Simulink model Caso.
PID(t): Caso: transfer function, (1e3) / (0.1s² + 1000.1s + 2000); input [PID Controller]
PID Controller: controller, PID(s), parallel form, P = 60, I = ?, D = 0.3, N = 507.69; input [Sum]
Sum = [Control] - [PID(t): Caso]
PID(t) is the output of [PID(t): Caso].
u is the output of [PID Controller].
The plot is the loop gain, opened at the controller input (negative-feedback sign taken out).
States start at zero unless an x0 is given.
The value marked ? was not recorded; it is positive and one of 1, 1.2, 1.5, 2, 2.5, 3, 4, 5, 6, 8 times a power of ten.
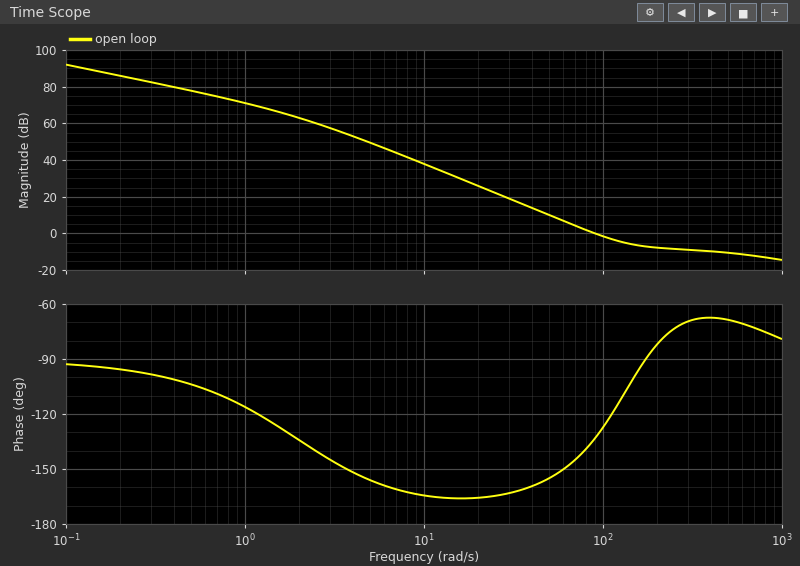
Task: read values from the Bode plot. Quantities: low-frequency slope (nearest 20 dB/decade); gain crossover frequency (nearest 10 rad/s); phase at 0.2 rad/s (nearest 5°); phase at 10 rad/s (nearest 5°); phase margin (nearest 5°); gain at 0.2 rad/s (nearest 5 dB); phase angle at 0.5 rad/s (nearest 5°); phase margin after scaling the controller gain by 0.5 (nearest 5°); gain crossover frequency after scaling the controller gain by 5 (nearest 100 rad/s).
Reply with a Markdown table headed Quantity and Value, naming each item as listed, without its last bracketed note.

| Quantity | Value |
|---|---|
| low-frequency slope | -20 dB/decade |
| gain crossover frequency | 90 rad/s |
| phase at 0.2 rad/s | -95° |
| phase at 10 rad/s | -165° |
| phase margin | 45° |
| gain at 0.2 rad/s | 85 dB |
| phase angle at 0.5 rad/s | -105° |
| phase margin after scaling the controller gain by 0.5 | 30° |
| gain crossover frequency after scaling the controller gain by 5 | 900 rad/s |
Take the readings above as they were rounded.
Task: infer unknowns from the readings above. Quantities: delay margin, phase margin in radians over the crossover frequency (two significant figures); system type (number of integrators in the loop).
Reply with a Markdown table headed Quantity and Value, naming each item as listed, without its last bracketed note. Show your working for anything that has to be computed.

| Quantity | Value |
|---|---|
| delay margin, phase margin in radians over the crossover frequency | 45 × π / 180 / 90 = 0.0087 s |
| system type | 1 |
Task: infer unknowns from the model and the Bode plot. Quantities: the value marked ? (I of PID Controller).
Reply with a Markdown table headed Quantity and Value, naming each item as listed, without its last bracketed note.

| Quantity | Value |
|---|---|
| the value marked ? | 8000 |
